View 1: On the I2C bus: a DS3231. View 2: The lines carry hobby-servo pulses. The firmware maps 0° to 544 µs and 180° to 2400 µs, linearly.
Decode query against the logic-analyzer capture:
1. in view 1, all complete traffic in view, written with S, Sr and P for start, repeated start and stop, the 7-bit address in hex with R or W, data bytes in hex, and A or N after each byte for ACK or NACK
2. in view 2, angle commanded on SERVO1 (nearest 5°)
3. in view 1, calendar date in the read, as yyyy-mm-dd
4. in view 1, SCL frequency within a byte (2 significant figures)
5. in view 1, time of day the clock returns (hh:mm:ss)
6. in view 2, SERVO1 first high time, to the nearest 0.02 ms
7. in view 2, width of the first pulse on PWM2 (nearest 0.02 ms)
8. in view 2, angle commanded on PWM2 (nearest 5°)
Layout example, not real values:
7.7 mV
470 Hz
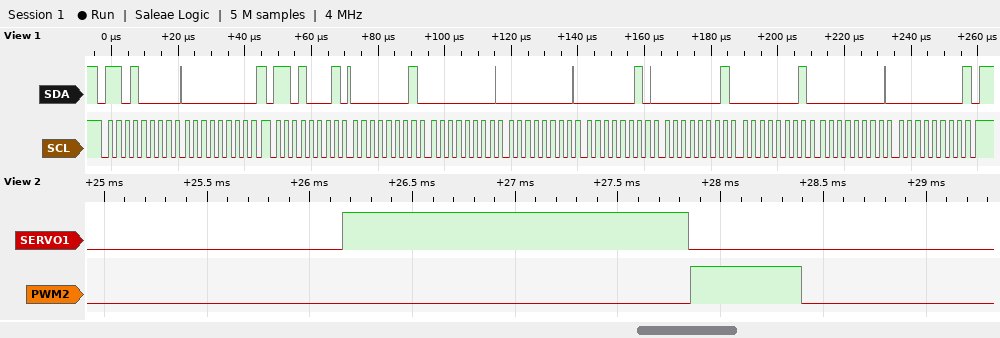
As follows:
S 68W A 00 A Sr 68R A 01 A 00 A 00 A 02 A 01 A 01 A 00 A 00 N P
110°
2000-01-01
400 kHz
00:00:01
1.68 ms
0.54 ms
0°
